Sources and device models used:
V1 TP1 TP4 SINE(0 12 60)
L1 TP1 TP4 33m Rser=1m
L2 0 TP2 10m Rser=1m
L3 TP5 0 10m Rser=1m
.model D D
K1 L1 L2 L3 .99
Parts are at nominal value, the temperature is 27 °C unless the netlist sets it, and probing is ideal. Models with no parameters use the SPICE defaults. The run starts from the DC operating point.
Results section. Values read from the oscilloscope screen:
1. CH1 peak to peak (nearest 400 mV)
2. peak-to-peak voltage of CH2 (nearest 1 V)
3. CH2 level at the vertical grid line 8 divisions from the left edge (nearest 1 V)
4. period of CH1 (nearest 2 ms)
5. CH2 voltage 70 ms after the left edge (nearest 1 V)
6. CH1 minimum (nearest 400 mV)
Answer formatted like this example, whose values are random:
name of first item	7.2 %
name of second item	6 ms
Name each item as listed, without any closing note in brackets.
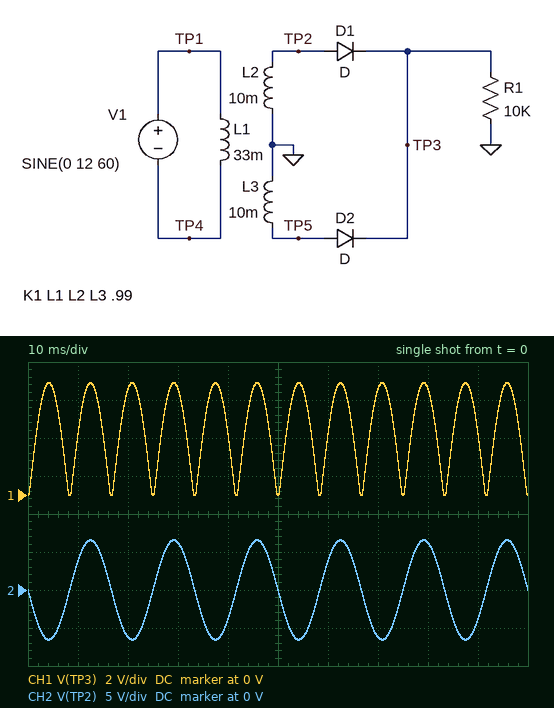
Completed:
CH1 peak to peak	6.0 V
peak-to-peak voltage of CH2	13 V
CH2 level at the vertical grid line 8 divisions from the left edge	6 V
period of CH1	8 ms
CH2 voltage 70 ms after the left edge	-6 V
CH1 minimum	0 V
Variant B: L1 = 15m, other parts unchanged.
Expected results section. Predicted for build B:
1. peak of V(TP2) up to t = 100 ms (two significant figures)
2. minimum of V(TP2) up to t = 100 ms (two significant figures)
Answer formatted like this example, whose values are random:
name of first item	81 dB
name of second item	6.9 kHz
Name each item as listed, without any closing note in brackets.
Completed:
peak of V(TP2) up to t = 100 ms	9.7 V
minimum of V(TP2) up to t = 100 ms	-9.7 V
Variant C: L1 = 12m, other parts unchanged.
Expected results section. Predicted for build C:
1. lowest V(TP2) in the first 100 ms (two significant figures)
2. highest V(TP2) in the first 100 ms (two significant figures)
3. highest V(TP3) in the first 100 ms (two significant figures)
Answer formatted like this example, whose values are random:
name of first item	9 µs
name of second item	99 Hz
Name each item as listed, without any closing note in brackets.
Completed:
lowest V(TP2) in the first 100 ms	-11 V
highest V(TP2) in the first 100 ms	11 V
highest V(TP3) in the first 100 ms	10 V
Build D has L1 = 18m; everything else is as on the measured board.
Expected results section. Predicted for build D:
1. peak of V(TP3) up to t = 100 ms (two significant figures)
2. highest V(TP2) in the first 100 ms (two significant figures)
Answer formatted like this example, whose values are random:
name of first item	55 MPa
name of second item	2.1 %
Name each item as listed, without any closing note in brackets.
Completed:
peak of V(TP3) up to t = 100 ms	8.2 V
highest V(TP2) in the first 100 ms	8.9 V
